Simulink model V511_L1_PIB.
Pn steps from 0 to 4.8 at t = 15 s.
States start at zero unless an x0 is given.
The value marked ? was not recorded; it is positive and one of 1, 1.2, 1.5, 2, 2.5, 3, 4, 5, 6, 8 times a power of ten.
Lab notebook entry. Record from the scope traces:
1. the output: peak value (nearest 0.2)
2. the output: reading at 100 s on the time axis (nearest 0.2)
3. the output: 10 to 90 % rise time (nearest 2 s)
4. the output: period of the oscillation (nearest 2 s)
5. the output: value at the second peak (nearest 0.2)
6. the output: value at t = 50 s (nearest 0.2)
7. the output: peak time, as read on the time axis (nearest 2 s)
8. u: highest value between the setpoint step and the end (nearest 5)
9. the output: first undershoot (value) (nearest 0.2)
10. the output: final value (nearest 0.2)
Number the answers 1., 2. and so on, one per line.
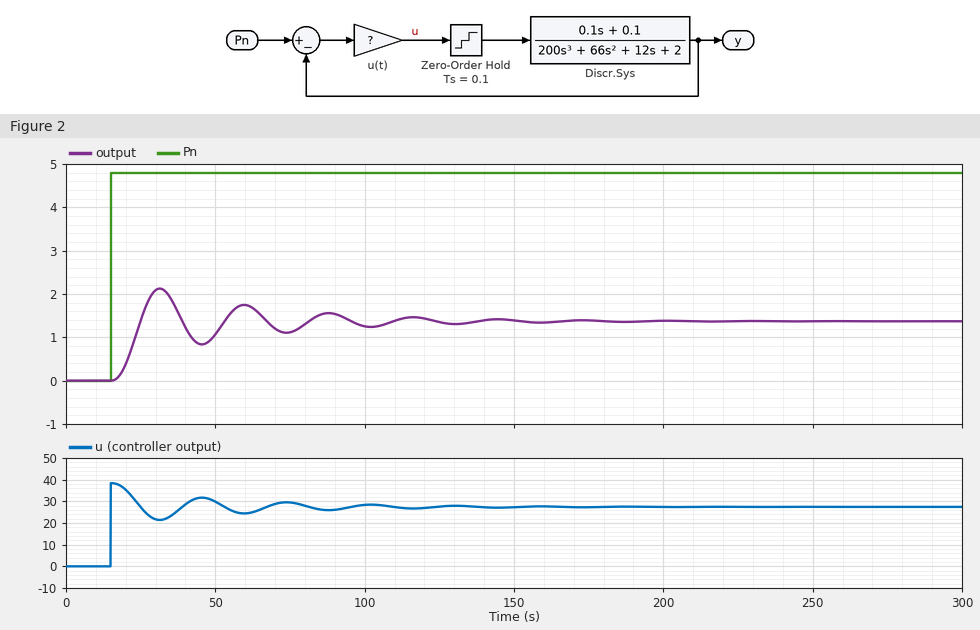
1. 2.2
2. 1.2
3. 6 s
4. 28 s
5. 1.8
6. 1.0
7. 32 s
8. 40
9. 0.8
10. 1.4
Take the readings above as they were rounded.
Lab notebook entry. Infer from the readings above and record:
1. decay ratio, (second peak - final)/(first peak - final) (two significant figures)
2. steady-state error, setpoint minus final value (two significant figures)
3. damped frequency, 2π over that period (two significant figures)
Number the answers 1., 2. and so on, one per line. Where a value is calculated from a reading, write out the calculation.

1. (1.8 - 1.4) / (2.2 - 1.4) = 0.50
2. 4.8 - 1.4 = 3.4
3. 2π / 28 = 0.22 rad/s
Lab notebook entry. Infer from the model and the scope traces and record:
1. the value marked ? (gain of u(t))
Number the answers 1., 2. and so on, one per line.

1. 8
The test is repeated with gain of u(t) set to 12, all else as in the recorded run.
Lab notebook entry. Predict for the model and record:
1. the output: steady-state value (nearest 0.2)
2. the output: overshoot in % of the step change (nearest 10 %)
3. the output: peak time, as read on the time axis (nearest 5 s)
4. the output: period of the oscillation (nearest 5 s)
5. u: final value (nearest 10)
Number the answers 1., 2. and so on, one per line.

1. 1.8
2. 60 %
3. 30 s
4. 25 s
5. 40
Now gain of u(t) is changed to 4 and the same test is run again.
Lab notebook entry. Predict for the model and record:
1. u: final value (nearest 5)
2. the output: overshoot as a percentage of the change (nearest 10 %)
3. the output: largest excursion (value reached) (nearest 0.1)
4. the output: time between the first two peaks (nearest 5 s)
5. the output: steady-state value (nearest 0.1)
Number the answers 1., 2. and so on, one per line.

1. 15
2. 50 %
3. 1.2
4. 30 s
5. 0.8
